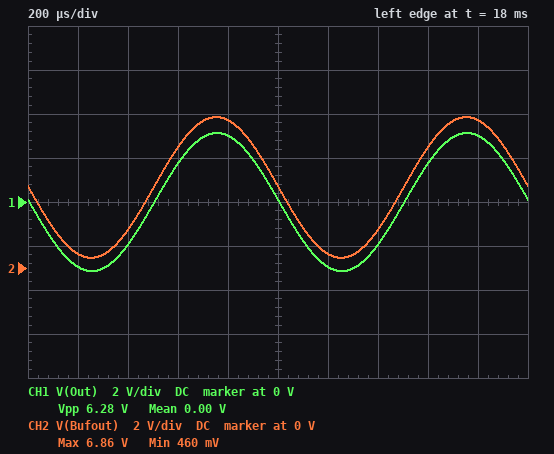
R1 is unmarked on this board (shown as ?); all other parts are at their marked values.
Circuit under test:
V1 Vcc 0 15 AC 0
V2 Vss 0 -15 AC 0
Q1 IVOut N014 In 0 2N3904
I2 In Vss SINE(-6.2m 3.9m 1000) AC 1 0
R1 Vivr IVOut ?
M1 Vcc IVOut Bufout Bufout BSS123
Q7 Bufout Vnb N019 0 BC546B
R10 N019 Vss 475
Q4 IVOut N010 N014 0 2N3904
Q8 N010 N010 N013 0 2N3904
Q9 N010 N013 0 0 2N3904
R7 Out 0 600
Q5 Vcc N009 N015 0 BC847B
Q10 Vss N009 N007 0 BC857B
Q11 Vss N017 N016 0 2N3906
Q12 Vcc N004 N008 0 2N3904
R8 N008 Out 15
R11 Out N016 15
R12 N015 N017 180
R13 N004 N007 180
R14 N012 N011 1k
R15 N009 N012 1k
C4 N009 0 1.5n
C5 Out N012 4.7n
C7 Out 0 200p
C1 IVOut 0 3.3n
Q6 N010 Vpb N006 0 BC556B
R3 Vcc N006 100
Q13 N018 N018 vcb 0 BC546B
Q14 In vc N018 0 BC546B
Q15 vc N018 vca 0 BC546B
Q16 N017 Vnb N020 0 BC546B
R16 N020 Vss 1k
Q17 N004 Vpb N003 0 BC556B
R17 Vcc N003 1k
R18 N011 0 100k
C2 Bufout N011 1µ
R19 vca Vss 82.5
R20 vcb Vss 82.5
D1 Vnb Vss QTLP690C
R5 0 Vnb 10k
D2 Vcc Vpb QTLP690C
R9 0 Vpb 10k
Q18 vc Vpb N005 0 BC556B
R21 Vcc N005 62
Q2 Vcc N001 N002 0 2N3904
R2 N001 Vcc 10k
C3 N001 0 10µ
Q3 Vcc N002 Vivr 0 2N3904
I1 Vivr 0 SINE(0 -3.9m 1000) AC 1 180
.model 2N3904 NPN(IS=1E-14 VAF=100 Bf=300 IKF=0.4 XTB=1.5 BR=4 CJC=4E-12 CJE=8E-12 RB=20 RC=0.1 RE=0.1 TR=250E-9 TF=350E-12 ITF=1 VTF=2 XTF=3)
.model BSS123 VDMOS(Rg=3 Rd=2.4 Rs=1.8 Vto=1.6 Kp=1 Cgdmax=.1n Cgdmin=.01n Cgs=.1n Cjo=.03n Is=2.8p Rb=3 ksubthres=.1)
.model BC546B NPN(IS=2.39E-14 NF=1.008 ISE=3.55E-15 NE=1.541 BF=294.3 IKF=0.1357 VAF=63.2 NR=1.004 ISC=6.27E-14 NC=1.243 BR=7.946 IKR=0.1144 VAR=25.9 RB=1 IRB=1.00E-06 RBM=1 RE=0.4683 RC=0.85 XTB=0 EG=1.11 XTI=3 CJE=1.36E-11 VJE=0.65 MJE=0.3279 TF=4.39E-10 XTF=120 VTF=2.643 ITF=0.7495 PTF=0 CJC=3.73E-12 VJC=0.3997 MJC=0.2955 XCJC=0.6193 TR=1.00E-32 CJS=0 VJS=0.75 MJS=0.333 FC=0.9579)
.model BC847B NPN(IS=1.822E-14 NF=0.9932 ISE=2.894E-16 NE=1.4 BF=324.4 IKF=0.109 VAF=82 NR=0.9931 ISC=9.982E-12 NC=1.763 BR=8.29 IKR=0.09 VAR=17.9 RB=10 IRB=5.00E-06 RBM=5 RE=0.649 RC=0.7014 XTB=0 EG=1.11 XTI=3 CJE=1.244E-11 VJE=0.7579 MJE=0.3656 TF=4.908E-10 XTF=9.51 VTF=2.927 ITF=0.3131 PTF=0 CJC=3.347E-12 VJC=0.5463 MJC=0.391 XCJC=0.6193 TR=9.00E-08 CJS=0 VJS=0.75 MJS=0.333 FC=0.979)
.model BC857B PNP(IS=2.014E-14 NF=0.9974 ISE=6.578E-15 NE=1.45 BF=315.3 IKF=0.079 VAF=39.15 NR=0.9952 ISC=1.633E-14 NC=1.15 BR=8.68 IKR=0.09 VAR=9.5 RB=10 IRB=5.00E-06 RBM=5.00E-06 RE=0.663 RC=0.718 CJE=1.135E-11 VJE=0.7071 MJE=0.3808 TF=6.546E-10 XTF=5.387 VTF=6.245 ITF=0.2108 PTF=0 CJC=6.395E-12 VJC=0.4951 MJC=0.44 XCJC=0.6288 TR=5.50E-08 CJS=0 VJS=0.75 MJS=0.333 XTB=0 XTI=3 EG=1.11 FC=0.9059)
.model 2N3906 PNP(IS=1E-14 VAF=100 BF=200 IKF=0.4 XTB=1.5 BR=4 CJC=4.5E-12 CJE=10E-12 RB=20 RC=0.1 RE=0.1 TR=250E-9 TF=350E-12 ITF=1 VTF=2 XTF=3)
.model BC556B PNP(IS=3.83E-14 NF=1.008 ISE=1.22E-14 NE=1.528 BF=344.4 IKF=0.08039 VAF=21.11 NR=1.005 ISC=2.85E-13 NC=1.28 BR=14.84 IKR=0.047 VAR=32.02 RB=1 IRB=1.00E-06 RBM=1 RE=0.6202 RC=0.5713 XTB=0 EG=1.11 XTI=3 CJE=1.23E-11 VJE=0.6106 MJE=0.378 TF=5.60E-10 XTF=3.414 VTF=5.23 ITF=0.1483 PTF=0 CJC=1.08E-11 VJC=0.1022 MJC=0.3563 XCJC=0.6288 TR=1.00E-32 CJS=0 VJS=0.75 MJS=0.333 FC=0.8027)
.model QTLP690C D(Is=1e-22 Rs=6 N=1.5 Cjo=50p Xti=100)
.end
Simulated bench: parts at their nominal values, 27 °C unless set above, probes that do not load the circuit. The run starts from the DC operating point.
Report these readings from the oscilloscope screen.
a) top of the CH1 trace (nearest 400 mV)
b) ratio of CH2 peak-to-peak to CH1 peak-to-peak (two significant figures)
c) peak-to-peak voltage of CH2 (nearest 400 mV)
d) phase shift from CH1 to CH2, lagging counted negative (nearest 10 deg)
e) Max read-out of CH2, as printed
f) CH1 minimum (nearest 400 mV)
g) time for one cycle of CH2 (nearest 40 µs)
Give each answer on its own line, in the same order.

3.2 V
1.0
6.4 V
0 deg
6.86 V
-3.2 V
1.00 ms
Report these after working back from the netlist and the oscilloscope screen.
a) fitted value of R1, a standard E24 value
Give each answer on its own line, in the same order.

820 Ω
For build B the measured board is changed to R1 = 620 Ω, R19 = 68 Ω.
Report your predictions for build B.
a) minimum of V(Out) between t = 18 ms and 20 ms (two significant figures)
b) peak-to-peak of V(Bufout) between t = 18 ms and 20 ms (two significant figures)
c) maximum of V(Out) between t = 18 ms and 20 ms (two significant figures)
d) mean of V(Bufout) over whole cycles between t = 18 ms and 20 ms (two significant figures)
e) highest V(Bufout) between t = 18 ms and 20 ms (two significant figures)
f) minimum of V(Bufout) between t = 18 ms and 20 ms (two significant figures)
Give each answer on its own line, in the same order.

-2.4 V
4.8 V
2.4 V
7.5 V
9.9 V
5.1 V
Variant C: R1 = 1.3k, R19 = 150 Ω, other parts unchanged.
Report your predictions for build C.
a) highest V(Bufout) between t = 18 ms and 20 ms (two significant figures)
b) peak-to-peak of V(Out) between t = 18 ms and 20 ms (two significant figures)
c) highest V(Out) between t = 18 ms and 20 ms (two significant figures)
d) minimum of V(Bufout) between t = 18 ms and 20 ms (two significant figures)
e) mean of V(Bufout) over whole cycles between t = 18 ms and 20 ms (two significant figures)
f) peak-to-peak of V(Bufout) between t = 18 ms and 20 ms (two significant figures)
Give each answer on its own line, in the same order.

-1.4 V
8.3 V
3.4 V
-9.8 V
-5.1 V
8.4 V
